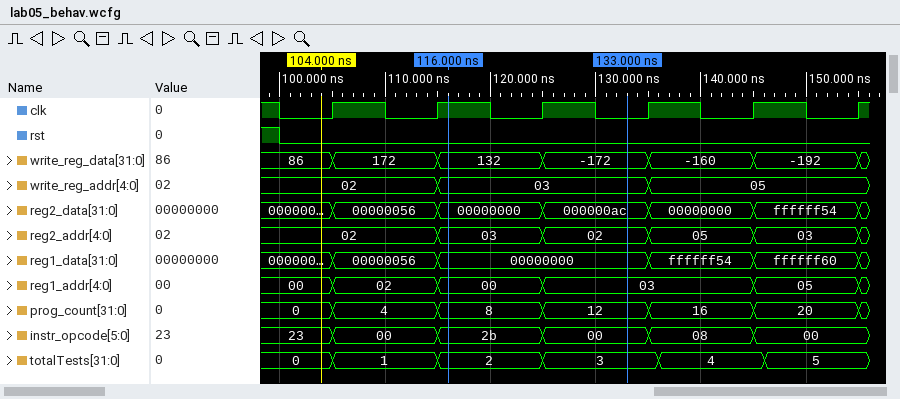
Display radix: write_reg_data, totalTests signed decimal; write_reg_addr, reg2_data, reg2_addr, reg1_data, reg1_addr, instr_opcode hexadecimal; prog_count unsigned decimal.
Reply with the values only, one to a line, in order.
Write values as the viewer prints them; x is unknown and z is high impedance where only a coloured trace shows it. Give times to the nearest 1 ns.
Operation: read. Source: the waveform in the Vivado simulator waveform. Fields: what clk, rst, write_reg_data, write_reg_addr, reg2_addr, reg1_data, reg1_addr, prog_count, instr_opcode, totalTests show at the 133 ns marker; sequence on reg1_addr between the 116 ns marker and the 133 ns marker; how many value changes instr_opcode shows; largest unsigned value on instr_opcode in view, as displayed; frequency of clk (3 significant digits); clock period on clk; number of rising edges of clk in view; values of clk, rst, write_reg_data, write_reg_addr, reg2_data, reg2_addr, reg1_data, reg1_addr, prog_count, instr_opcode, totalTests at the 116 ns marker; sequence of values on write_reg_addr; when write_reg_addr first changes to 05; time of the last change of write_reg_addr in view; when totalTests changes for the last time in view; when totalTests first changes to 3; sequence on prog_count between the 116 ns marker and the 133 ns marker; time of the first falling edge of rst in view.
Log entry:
clk=0, rst=0, write_reg_data=-172, write_reg_addr=03, reg2_addr=02, reg1_data=00000000, reg1_addr=03, prog_count=12, instr_opcode=00, totalTests=3
00, 03
5
2b
100 MHz
10 ns
6
clk=1, rst=0, write_reg_data=132, write_reg_addr=03, reg2_data=00000000, reg2_addr=03, reg1_data=00000000, reg1_addr=00, prog_count=8, instr_opcode=2b, totalTests=2
02, 03, 05
135 ns
135 ns
146 ns
125 ns
8, 12
100 ns
